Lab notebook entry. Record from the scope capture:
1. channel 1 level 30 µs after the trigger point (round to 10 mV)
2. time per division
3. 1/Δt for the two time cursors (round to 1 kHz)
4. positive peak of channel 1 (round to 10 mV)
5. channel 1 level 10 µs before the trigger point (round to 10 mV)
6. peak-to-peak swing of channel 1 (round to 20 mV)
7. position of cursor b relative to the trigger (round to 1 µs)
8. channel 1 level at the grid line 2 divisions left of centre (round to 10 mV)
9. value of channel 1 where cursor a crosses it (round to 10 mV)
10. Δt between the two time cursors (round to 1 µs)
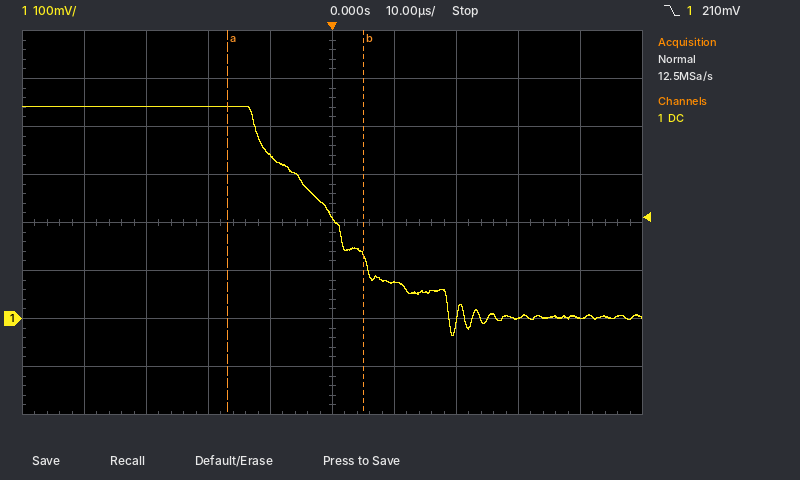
0 mV
10 µs
45 kHz
440 mV
340 mV
480 mV
+5 µs
440 mV
440 mV
22 µs
